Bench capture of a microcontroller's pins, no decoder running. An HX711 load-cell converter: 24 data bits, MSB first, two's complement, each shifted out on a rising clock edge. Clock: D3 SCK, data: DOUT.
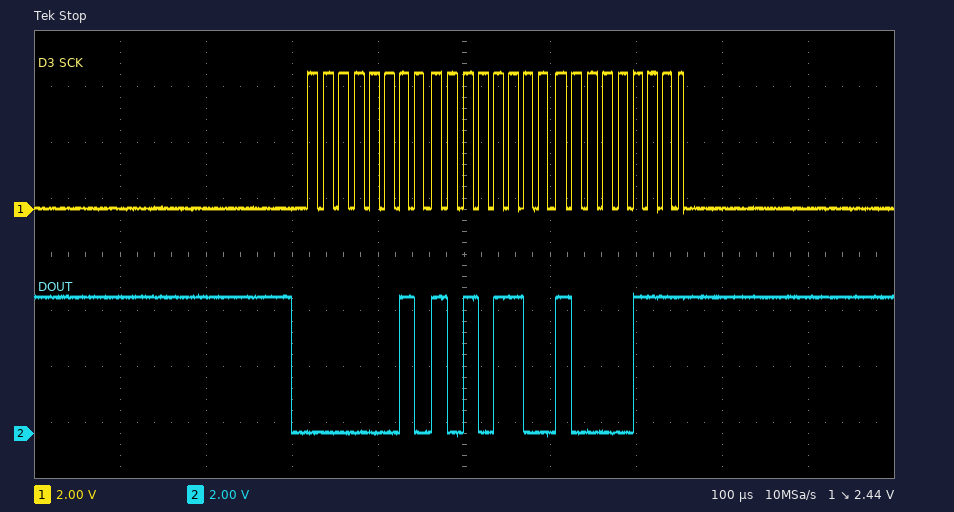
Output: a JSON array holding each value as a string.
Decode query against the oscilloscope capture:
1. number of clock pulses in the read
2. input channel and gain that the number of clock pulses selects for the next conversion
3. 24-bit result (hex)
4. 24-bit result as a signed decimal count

["25", "channel A, gain 128", "0x02AC87", "175239"]
